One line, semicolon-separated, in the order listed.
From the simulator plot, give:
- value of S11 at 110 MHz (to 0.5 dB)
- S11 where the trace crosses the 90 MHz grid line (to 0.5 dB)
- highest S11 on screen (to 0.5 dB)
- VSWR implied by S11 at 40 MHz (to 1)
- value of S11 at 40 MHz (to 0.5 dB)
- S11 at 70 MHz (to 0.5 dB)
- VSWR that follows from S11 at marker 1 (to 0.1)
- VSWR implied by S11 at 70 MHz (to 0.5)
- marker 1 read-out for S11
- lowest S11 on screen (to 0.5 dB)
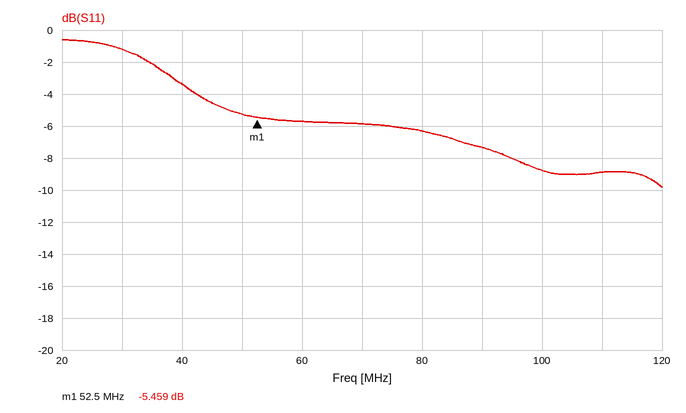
-9.0 dB; -7.5 dB; -0.5 dB; 5; -3.5 dB; -6.0 dB; 3.3; 3.0; -5.459 dB; -10.0 dB
